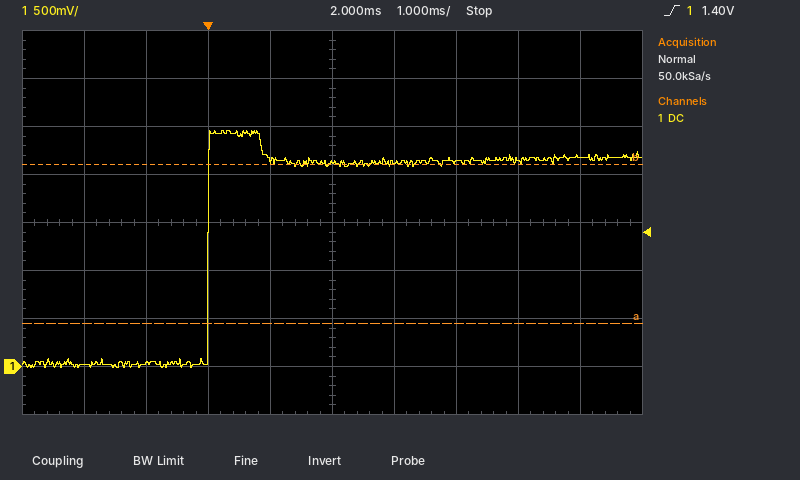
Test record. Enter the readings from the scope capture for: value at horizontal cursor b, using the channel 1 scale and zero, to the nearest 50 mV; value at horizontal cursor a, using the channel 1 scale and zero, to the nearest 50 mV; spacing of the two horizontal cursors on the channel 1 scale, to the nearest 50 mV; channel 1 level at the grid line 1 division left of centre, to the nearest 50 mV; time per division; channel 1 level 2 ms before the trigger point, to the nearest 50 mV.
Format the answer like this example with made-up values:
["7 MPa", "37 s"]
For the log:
["2.10 V", "450 mV", "1.65 V", "2.15 V", "1 ms", "0 mV"]
